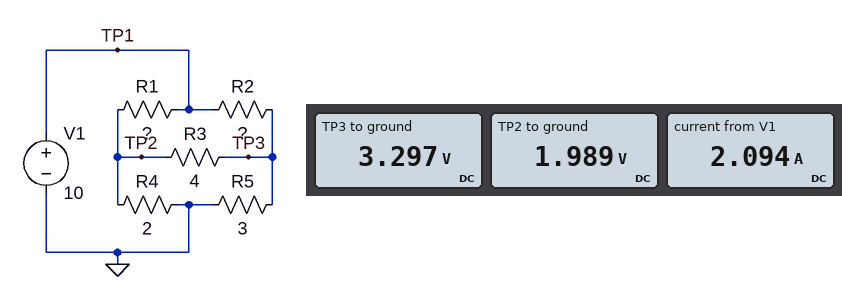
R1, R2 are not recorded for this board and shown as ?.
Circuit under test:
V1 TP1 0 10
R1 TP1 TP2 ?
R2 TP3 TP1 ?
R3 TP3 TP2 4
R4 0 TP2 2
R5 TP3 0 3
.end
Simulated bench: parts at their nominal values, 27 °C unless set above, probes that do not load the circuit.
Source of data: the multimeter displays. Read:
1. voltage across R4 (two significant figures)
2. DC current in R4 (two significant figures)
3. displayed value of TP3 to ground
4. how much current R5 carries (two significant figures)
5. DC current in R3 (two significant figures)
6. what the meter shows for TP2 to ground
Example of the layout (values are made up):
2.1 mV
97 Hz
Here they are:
2.0 V
990 mA
3.297 V
1.1 A
330 mA
1.989 V
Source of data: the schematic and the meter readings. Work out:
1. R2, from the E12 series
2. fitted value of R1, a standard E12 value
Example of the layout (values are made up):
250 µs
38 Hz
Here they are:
4.7 Ω
12 Ω
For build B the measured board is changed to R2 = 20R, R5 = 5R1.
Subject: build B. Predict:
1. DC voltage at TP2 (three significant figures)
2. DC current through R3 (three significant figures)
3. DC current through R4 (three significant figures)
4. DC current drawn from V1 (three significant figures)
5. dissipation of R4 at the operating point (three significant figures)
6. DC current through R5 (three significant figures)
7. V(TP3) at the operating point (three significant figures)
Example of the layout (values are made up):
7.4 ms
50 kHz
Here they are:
1.53 V
61.7 mA
767 mA
1.12 A
1.18 W
349 mA
1.78 V
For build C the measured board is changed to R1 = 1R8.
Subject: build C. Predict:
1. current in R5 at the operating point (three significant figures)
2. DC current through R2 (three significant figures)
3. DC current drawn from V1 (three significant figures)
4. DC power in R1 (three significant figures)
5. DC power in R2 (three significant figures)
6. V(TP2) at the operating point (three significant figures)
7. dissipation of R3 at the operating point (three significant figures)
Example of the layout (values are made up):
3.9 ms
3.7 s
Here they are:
1.42 A
1.22 A
3.96 A
13.5 W
7.00 W
5.07 V
163 mW
